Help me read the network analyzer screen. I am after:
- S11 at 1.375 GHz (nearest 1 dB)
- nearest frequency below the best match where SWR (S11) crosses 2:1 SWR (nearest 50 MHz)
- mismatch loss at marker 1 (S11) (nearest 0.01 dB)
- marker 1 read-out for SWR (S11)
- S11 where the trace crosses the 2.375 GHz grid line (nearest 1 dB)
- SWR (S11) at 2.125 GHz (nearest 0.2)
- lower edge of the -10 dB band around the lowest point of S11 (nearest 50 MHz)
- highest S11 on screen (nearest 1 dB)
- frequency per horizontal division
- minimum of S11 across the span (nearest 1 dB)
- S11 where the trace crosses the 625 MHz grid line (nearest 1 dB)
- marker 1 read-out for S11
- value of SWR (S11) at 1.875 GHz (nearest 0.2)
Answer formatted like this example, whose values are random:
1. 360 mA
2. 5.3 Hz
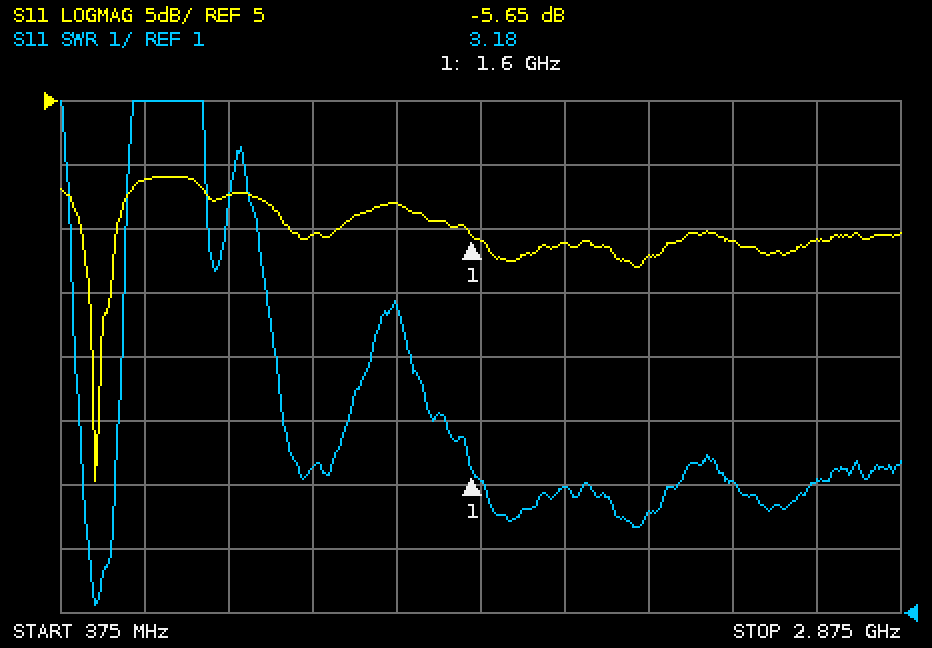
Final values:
1. -3 dB
2. 450 MHz
3. 1.38 dB
4. 3.18
5. -6 dB
6. 2.6
7. 450 MHz
8. -1 dB
9. 250 MHz
10. -25 dB
11. -1 dB
12. -5.65 dB
13. 3.0
